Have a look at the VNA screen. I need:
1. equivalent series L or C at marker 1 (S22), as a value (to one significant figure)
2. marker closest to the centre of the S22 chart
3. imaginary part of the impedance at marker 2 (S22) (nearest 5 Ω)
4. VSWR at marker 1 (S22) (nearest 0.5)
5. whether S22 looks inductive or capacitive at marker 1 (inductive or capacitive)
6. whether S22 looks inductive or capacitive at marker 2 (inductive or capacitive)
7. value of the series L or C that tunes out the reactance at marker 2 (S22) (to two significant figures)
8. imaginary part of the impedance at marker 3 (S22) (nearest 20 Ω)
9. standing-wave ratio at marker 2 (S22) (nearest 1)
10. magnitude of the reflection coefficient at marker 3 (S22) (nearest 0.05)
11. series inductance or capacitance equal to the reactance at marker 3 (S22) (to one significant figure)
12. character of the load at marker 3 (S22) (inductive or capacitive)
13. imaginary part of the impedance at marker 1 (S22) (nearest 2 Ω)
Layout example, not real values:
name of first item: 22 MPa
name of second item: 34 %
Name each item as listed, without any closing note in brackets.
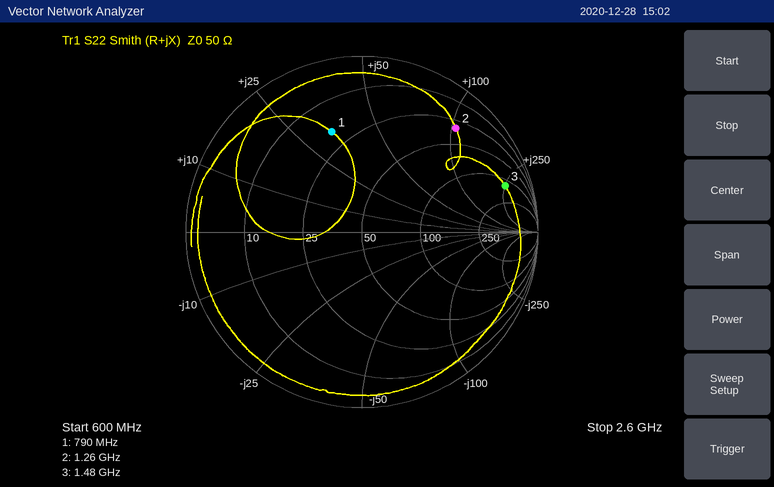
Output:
equivalent series L or C at marker 1 (S22), as a value: 7 nH
marker closest to the centre of the S22 chart: marker 1
imaginary part of the impedance at marker 2 (S22): +105 Ω
VSWR at marker 1 (S22): 4.0
whether S22 looks inductive or capacitive at marker 1: inductive
whether S22 looks inductive or capacitive at marker 2: inductive
value of the series L or C that tunes out the reactance at marker 2 (S22): 1.2 pF
imaginary part of the impedance at marker 3 (S22): +260 Ω
standing-wave ratio at marker 2 (S22): 9
magnitude of the reflection coefficient at marker 3 (S22): 0.85
series inductance or capacitance equal to the reactance at marker 3 (S22): 30 nH
character of the load at marker 3 (S22): inductive
imaginary part of the impedance at marker 1 (S22): +34 Ω
